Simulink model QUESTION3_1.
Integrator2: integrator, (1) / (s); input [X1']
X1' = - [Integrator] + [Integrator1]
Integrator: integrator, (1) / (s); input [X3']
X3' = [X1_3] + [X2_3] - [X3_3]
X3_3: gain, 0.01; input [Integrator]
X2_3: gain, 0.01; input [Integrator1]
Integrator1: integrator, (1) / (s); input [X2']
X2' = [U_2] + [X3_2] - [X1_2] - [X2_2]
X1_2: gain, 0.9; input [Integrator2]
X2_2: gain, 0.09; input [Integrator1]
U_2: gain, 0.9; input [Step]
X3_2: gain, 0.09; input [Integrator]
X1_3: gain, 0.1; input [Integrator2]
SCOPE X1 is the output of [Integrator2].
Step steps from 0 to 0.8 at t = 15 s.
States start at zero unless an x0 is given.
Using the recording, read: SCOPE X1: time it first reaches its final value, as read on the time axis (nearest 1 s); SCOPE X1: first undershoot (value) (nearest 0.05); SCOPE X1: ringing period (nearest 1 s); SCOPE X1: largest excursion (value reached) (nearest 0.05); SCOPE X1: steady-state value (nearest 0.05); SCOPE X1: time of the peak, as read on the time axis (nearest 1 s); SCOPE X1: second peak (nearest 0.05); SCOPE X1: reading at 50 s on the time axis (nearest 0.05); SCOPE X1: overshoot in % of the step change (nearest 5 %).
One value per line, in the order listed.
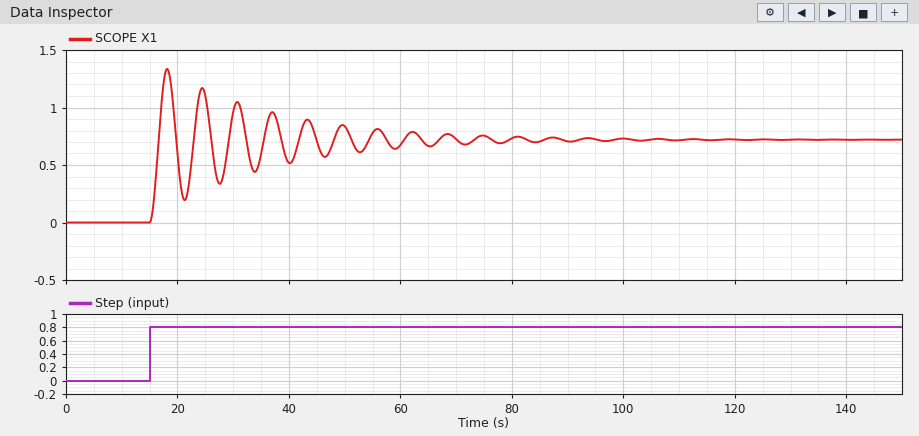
17 s
0.20
6 s
1.35
0.70
18 s
1.15
0.85
85 %
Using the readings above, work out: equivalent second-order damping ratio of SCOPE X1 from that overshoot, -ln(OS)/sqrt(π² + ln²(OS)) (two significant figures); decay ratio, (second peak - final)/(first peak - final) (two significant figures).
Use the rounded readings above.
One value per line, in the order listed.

0.052
0.69
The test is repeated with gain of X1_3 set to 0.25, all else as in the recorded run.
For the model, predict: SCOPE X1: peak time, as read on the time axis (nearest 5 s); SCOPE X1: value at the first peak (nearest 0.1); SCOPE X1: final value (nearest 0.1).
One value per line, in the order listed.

20 s
1.2
0.6
